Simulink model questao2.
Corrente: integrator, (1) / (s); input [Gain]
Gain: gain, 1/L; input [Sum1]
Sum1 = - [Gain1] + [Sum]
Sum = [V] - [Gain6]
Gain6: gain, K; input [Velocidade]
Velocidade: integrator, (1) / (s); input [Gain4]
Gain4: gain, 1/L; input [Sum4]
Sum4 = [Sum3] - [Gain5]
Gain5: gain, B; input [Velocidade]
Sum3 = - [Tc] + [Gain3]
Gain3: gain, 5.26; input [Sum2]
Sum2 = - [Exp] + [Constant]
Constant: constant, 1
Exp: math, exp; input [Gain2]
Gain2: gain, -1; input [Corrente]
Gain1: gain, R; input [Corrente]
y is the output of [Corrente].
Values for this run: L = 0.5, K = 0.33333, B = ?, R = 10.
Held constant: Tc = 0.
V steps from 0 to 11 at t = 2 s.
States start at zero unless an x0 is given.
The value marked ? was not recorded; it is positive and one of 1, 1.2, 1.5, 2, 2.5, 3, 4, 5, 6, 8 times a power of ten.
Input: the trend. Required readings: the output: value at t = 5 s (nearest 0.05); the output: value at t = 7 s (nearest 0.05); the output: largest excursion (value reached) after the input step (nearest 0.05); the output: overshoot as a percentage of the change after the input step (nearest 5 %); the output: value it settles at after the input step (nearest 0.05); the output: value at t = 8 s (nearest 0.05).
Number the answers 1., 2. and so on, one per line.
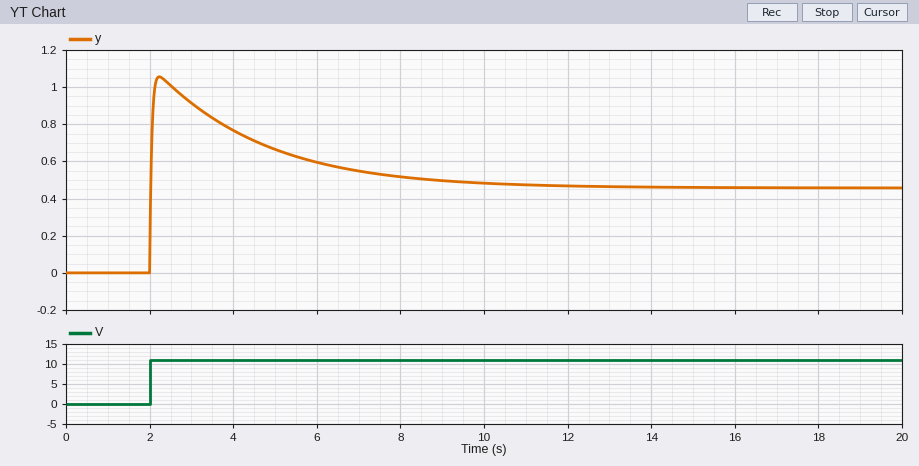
1. 0.65
2. 0.55
3. 1.05
4. 130 %
5. 0.45
6. 0.50
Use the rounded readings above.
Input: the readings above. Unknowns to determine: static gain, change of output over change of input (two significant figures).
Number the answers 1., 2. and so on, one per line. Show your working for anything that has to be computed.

1. (0.45 - 0) / (11 - 0) = 0.041
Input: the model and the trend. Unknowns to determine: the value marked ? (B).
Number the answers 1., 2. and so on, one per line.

1. 0.1
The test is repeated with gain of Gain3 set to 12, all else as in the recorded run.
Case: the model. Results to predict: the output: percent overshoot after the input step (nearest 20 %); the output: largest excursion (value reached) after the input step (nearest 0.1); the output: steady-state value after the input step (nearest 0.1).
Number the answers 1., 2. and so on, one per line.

1. 320 %
2. 1.0
3. 0.2
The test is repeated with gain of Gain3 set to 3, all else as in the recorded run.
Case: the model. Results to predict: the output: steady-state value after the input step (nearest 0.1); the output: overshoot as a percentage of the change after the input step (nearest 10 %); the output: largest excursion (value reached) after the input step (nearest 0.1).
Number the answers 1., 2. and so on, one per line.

1. 0.6
2. 70 %
3. 1.1
